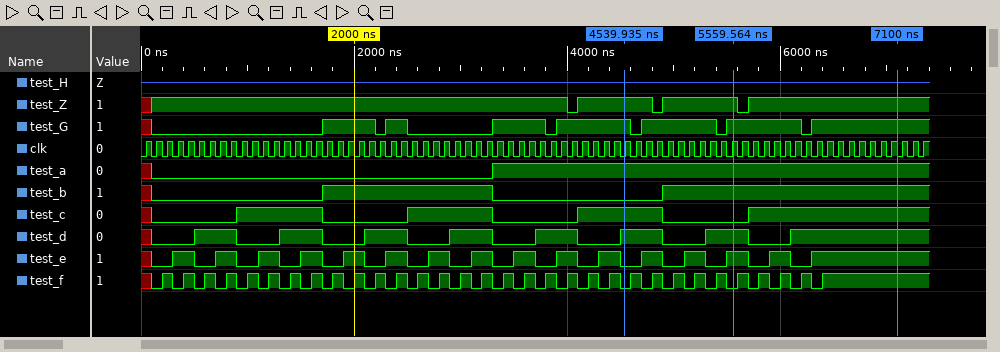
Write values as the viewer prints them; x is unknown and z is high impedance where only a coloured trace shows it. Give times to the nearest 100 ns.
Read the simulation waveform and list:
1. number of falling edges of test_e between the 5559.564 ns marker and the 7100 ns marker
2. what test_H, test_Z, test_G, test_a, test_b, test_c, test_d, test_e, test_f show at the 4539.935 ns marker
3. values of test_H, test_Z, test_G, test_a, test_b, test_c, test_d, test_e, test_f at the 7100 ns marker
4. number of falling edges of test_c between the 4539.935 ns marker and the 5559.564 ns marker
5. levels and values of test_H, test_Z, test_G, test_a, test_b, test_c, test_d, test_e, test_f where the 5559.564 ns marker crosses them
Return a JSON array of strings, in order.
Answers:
["2", "test_H=z, test_Z=1, test_G=1, test_a=1, test_b=0, test_c=1, test_d=1, test_e=0, test_f=0", "test_H=z, test_Z=1, test_G=1, test_a=1, test_b=1, test_c=1, test_d=1, test_e=1, test_f=1", "1", "test_H=z, test_Z=1, test_G=1, test_a=1, test_b=1, test_c=0, test_d=1, test_e=1, test_f=0"]
